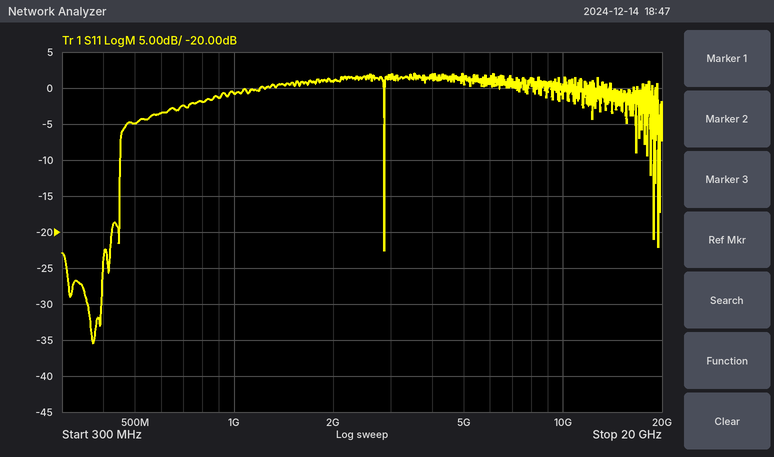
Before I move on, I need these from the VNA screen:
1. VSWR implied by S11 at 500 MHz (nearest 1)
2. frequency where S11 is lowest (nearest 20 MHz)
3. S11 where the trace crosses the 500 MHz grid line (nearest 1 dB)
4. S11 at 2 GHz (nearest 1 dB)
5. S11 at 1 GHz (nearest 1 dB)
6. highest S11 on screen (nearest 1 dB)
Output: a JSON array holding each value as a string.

["4", "380 MHz", "-5 dB", "1 dB", "-1 dB", "2 dB"]
